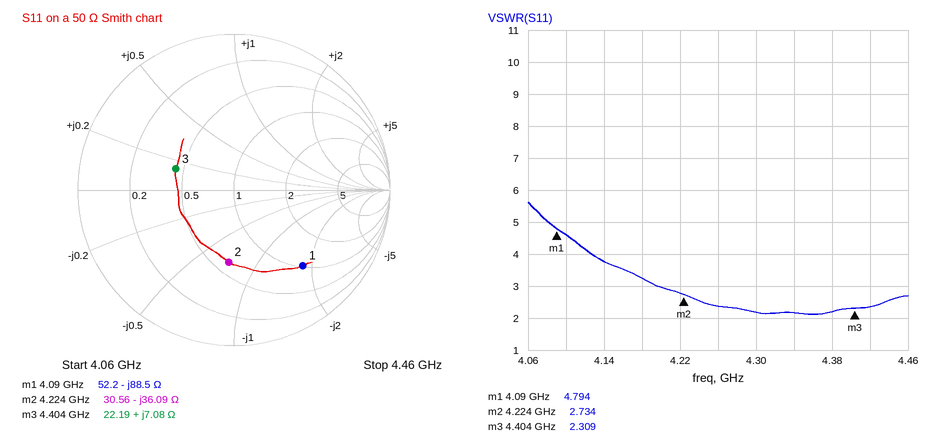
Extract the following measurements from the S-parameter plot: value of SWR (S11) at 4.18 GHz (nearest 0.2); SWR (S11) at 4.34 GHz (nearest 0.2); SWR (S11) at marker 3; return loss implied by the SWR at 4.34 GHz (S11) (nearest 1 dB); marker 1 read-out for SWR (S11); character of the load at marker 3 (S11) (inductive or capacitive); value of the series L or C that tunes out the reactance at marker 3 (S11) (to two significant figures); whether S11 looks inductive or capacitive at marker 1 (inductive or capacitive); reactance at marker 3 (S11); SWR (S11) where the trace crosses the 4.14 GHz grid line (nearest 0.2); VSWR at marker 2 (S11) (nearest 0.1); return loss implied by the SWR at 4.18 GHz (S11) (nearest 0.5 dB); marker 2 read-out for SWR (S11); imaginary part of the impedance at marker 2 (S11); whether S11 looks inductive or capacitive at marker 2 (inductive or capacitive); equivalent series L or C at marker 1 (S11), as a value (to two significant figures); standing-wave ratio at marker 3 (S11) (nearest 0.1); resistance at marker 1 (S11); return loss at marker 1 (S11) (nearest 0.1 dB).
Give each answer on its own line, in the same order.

3.2
2.2
2.309
9 dB
4.794
inductive
5.1 pF
capacitive
+7.08 Ω
3.8
2.7
5.5 dB
2.734
-36.09 Ω
capacitive
440 fF
2.3
52.2 Ω
3.7 dB
